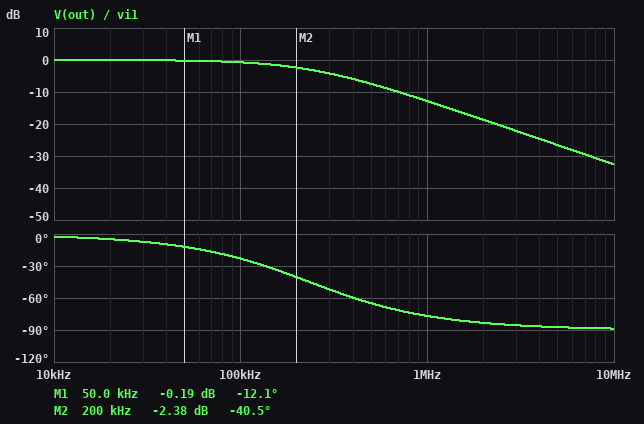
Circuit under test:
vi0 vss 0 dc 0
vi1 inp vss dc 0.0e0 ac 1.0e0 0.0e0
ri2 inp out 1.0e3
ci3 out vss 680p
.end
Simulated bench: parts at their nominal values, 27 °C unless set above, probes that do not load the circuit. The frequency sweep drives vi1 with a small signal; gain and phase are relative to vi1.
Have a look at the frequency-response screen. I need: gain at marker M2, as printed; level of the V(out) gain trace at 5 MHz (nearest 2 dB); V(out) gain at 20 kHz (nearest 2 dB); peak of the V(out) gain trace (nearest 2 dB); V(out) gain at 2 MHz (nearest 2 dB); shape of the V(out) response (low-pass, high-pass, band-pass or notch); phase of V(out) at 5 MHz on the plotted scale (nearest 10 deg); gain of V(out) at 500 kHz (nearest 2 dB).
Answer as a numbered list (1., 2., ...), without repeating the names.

1. -2.38 dB
2. -26 dB
3. 0 dB
4. 0 dB
5. -18 dB
6. low-pass
7. -90 deg
8. -8 dB
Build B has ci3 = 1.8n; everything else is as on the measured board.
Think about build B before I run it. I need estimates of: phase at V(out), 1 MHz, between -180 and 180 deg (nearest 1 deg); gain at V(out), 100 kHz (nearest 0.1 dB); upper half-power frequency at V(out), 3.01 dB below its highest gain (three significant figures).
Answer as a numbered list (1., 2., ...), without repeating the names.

1. -85 deg
2. -3.6 dB
3. 88.4 kHz
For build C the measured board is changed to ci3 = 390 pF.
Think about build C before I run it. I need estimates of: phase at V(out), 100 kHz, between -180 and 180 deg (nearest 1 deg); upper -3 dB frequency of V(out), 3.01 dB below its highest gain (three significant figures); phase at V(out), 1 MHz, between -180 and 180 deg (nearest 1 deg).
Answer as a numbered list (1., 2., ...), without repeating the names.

1. -14 deg
2. 408 kHz
3. -68 deg
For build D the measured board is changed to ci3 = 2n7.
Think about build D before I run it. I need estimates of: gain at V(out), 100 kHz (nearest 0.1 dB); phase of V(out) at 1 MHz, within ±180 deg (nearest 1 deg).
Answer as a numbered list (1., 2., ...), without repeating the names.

1. -5.9 dB
2. -87 deg
